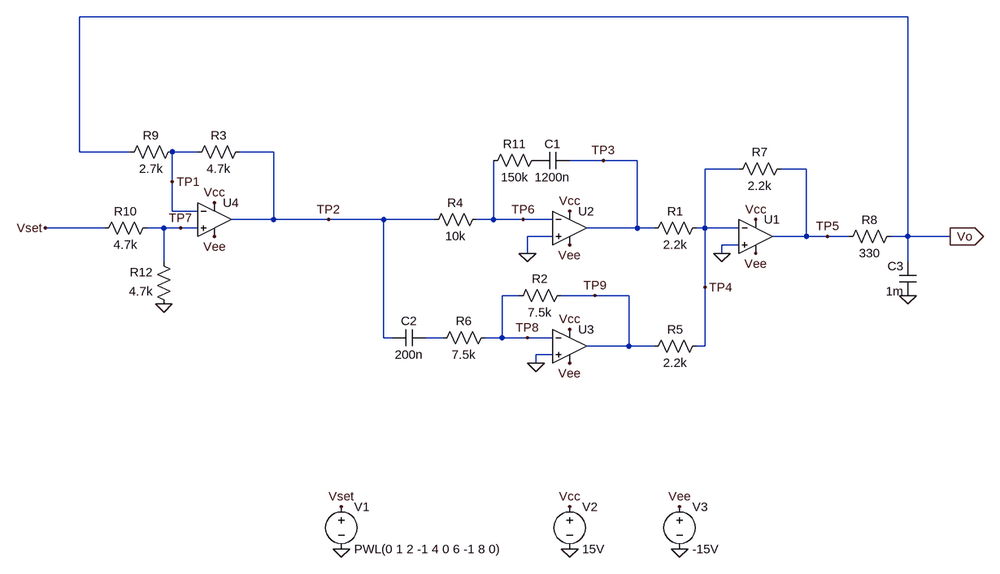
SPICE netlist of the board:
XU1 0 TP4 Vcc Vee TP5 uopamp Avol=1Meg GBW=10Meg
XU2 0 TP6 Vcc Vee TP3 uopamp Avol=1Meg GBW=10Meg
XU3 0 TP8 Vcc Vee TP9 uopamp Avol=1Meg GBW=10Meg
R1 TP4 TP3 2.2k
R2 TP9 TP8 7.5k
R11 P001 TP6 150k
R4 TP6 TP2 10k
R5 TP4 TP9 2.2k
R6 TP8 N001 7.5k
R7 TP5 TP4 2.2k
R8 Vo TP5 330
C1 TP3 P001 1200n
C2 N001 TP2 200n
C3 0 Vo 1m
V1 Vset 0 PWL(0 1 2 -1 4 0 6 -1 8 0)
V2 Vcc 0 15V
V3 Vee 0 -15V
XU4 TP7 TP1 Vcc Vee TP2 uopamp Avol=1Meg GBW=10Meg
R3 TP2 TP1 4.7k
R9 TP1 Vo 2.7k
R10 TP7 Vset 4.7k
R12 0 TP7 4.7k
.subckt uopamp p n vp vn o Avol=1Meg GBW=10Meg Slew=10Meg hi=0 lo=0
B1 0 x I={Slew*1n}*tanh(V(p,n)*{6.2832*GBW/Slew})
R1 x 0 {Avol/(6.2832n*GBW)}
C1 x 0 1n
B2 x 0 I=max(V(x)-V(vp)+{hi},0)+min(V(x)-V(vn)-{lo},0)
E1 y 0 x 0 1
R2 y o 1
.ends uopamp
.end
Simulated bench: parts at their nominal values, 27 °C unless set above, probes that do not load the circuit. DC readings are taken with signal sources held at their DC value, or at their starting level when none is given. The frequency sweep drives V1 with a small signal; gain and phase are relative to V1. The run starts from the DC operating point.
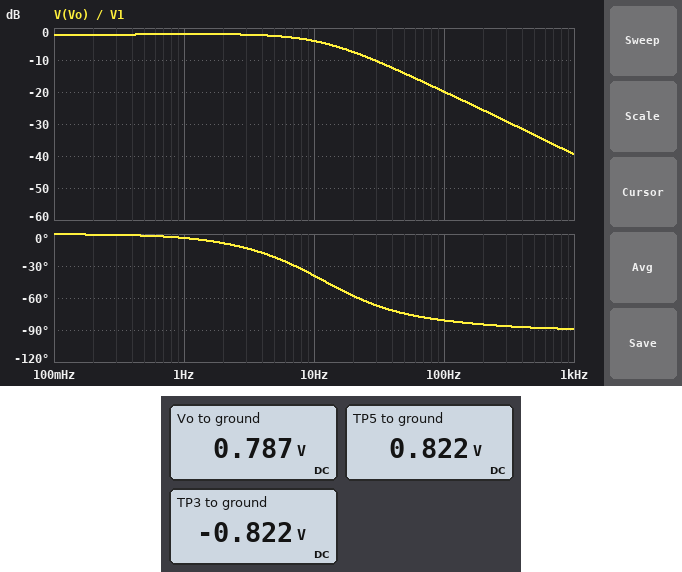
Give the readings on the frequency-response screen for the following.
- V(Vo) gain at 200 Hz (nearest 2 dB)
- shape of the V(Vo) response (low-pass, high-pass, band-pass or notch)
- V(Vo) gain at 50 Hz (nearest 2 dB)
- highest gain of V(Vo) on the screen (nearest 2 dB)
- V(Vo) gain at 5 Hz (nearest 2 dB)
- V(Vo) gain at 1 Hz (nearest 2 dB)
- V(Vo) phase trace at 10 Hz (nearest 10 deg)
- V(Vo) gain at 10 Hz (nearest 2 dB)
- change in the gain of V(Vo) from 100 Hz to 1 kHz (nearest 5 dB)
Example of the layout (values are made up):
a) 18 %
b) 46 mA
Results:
a) -26 dB
b) low-pass
c) -14 dB
d) -2 dB
e) -2 dB
f) -2 dB
g) -40 deg
h) -4 dB
i) -20 dB
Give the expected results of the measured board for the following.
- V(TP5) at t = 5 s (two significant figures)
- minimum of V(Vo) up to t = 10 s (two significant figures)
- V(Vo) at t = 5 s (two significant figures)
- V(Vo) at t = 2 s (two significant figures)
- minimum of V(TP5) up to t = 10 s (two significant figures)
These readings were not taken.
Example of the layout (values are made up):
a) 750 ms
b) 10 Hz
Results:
a) -540 mV
b) -790 mV
c) -390 mV
d) -780 mV
e) -1.1 V
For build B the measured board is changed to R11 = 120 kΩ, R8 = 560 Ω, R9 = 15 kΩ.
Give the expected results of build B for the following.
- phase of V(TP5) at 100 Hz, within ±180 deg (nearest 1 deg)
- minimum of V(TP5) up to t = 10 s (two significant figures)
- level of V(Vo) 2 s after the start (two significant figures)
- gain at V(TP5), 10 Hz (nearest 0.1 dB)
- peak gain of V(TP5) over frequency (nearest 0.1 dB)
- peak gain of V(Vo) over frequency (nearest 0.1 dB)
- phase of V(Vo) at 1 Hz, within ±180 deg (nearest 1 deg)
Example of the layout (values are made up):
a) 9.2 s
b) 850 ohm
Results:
a) 2 deg
b) -3.2 V
c) -2.0 V
d) 18.0 dB
e) 19.8 dB
f) 8.0 dB
g) -40 deg
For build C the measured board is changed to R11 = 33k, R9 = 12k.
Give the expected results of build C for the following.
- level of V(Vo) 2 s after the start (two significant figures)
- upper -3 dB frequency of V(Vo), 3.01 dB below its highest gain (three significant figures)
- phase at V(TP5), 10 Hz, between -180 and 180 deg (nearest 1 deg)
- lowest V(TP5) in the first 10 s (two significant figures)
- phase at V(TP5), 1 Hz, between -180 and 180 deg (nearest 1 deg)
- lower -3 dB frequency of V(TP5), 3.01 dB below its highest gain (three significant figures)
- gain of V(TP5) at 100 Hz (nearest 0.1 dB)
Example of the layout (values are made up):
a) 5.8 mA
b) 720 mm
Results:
a) -1.7 V
b) 1.92 Hz
c) -17 deg
d) -2.3 V
e) 41 deg
f) 1.11 Hz
g) 8.4 dB
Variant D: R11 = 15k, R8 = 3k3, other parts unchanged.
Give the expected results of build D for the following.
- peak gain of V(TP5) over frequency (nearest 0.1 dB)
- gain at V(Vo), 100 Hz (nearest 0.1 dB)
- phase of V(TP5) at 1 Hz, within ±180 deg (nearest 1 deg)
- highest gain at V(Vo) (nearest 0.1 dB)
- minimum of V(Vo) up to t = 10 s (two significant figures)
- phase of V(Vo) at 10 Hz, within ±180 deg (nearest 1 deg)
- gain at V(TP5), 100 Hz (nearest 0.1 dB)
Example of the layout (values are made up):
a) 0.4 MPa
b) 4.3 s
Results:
a) 37.9 dB
b) -55.8 dB
c) 28 deg
d) 11.2 dB
e) -840 mV
f) -121 deg
g) 8.8 dB
